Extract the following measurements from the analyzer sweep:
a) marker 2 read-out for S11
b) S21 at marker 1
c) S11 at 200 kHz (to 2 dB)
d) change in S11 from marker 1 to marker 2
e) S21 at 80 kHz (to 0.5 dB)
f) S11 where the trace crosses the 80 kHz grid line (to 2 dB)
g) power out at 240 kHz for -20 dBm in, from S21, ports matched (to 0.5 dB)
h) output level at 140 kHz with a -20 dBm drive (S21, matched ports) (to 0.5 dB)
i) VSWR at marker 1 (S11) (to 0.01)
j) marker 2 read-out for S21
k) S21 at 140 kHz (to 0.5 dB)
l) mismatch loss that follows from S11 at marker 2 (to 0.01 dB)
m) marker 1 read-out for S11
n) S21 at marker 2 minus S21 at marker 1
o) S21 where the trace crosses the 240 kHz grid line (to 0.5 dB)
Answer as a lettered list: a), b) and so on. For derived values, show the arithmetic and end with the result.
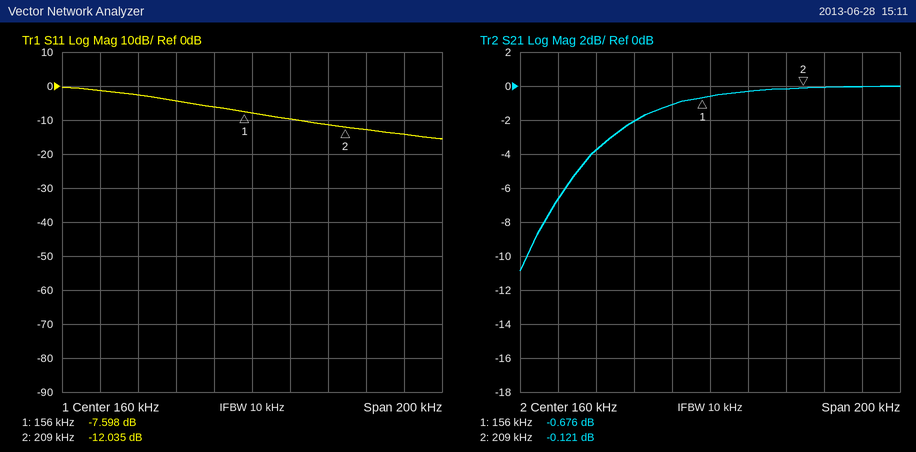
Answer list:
a) -12.035 dB
b) -0.676 dB
c) -12 dB
d) -12.035 − (-7.598) = -4.437 dB
e) -6.5 dB
f) -2 dB
g) -20 dBm + (0.0 dB) = -20.0 dBm
h) -20 dBm + (-1.0 dB) = -21.0 dBm
i) (1 + 0.4170)/(1 − 0.4170) ≈ 2.43
j) -0.121 dB
k) -1.0 dB
l) −10 log10(1 − 10^(-12.035/10)) ≈ 0.28 dB
m) -7.598 dB
n) -0.121 − (-0.676) = 0.555 dB
o) 0.0 dB
